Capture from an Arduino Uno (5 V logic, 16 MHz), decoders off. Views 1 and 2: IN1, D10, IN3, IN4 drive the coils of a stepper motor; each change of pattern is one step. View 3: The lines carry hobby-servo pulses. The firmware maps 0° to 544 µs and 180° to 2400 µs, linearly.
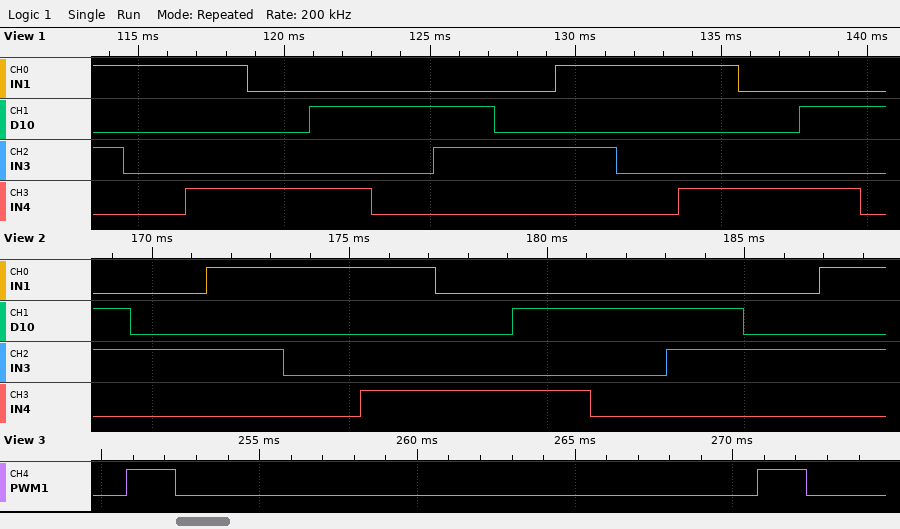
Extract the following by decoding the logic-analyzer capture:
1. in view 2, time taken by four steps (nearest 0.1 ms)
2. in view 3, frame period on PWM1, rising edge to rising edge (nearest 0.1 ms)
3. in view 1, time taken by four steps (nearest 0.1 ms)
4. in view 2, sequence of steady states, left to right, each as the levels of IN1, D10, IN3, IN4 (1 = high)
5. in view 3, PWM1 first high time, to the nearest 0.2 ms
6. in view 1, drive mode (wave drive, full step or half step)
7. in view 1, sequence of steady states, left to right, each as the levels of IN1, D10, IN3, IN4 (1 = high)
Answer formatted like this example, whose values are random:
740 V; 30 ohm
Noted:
7.7 ms; 20.0 ms; 8.5 ms; 0110 0010 1010 1000 1001 0001 0101 0100 0110 0010 1010; 1.6 ms; half step; 1010 1000 1001 0001 0101 0100 0110 0010 1010 1000 1001 0001 0101 0100
